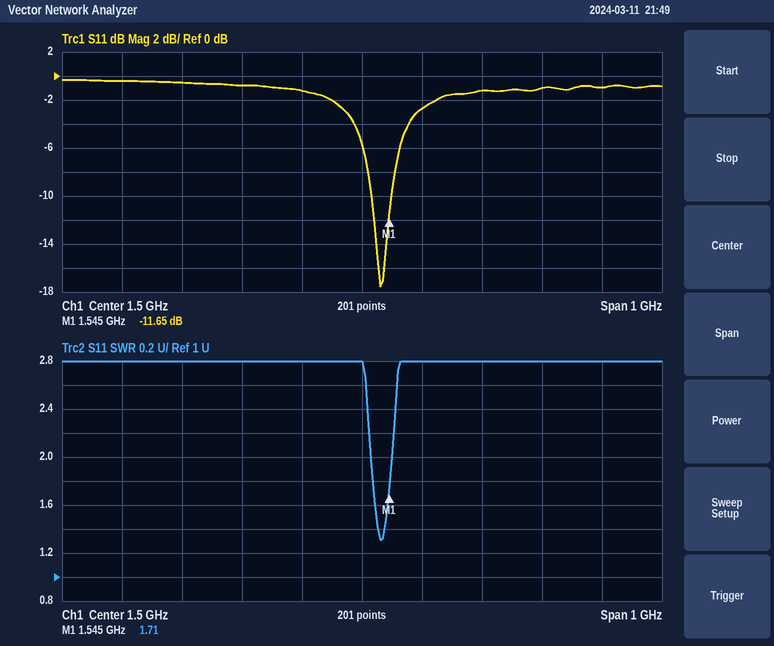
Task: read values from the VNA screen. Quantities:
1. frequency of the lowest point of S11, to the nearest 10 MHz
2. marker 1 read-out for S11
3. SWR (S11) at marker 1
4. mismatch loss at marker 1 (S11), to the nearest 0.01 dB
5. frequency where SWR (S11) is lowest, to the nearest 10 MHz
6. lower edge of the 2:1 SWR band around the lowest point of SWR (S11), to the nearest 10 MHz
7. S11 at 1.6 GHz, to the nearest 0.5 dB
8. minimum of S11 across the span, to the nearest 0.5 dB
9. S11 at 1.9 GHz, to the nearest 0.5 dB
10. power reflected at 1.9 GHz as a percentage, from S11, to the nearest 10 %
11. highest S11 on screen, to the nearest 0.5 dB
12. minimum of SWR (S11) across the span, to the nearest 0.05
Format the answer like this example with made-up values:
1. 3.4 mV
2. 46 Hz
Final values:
1. 1.53 GHz
2. -11.65 dB
3. 1.71
4. 0.31 dB
5. 1.53 GHz
6. 1.51 GHz
7. -2.5 dB
8. -17.5 dB
9. -1.0 dB
10. 80 %
11. -0.5 dB
12. 1.30
